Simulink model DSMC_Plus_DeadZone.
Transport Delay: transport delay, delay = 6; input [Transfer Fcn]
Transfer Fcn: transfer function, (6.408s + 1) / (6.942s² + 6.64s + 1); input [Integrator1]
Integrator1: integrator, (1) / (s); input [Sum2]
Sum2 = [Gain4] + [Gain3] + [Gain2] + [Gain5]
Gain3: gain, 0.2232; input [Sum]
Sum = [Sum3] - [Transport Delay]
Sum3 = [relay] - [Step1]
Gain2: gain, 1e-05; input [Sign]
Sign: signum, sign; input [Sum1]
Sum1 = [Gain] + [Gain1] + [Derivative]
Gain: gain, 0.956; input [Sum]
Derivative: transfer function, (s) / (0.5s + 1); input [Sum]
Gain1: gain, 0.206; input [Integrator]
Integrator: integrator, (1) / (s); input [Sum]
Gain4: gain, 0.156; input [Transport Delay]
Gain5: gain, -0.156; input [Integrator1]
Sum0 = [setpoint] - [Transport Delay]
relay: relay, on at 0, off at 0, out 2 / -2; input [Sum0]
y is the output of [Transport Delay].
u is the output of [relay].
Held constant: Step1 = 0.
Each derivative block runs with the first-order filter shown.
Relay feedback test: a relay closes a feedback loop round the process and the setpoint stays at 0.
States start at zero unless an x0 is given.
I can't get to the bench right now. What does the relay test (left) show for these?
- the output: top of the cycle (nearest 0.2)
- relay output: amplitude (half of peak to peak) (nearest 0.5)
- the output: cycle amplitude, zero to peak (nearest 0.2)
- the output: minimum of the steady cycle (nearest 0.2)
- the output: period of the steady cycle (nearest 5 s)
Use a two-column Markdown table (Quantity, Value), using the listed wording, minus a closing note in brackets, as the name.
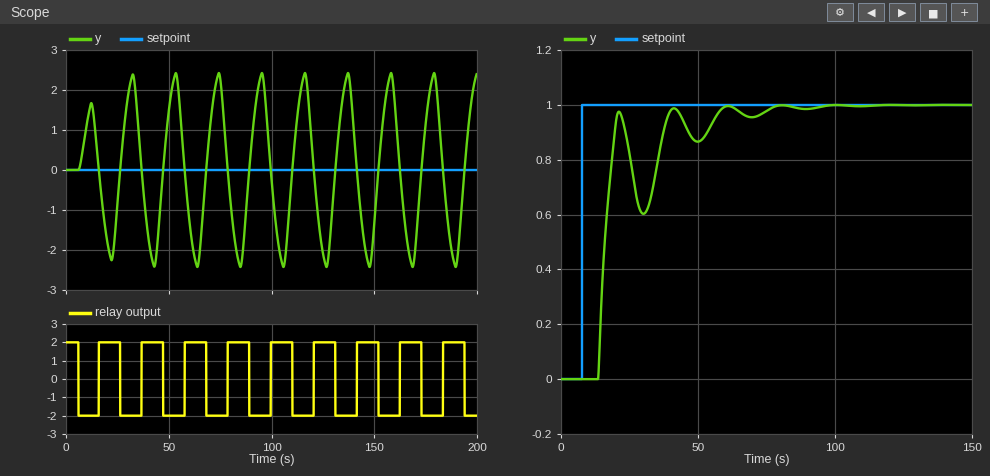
| Quantity | Value |
|---|---|
| the output: top of the cycle | 2.4 |
| relay output: amplitude (half of peak to peak) | 2.0 |
| the output: cycle amplitude, zero to peak | 2.4 |
| the output: minimum of the steady cycle | -2.4 |
| the output: period of the steady cycle | 20 s |
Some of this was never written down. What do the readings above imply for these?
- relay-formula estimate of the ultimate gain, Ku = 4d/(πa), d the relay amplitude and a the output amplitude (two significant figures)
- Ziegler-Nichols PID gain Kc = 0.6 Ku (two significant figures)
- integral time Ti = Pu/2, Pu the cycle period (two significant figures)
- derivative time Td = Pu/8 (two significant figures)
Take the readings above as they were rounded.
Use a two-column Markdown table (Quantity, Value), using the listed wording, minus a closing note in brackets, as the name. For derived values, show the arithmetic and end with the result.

| Quantity | Value |
|---|---|
| relay-formula estimate of the ultimate gain, Ku = 4d/(πa), d the relay amplitude and a the output amplitude | 4 × 2 / (π × 2.4) = 1.1 |
| Ziegler-Nichols PID gain Kc = 0.6 Ku | 0.6 × 1.1 = 0.66 |
| integral time Ti = Pu/2, Pu the cycle period | 20 / 2 = 10 s |
| derivative time Td = Pu/8 | 20 / 8 = 2.5 s |
